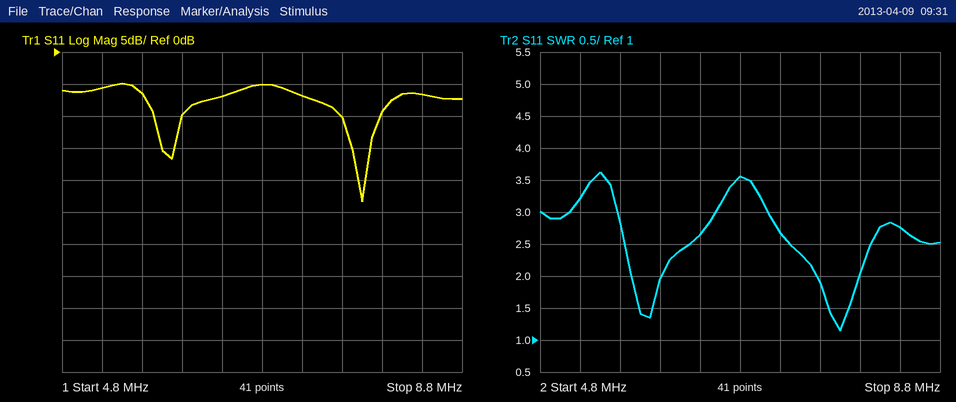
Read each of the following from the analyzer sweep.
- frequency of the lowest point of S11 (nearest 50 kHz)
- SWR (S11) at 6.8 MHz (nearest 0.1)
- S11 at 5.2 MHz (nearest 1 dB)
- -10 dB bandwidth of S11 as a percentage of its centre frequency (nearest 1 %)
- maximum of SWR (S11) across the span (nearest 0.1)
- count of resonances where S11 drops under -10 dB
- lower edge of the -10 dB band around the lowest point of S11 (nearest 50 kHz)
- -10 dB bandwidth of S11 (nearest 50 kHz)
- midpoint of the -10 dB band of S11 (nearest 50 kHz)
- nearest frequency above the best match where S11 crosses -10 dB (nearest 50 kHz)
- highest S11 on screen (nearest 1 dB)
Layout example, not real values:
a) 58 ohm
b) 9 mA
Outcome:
a) 7.80 MHz
b) 3.6
c) -6 dB
d) 5 %
e) 3.6
f) 2
g) 7.60 MHz
h) 400 kHz
i) 7.80 MHz
j) 8.00 MHz
k) -5 dB
